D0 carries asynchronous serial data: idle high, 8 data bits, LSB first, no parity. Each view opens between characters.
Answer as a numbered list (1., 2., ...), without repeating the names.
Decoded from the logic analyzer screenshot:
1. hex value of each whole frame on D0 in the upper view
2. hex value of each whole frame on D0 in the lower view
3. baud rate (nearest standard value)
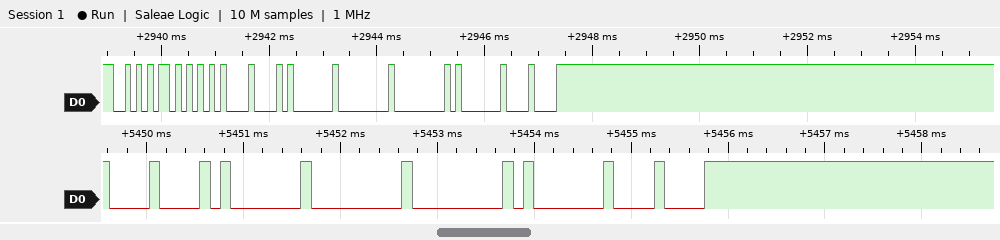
1. AA, 55, 08, 01, 00, 00, 01, 08
2. 08, 01, 00, 00, 01, 08
3. 9600 baud
